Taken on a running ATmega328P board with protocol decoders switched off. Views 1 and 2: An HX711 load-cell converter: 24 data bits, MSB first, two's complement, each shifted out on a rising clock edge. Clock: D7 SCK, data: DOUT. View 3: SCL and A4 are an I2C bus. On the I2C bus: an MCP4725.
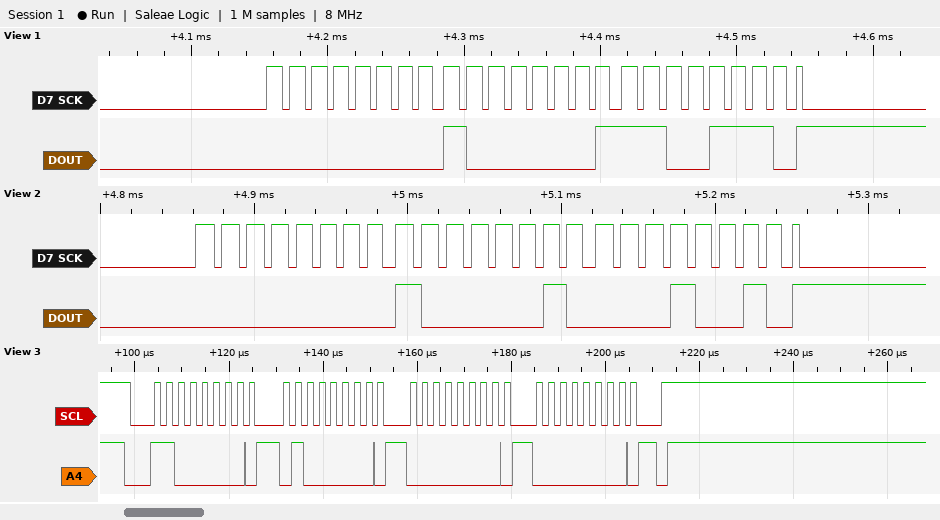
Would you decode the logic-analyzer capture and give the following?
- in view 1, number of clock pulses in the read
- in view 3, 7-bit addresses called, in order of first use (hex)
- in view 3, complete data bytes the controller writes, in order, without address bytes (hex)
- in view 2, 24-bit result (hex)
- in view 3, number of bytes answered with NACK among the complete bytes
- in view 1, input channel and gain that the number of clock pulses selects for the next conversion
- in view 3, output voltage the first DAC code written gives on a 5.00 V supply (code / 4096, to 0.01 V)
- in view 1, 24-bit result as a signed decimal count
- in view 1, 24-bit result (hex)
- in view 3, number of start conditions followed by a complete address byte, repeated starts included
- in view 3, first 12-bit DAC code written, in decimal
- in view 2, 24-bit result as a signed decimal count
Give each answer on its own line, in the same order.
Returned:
25
0x60
40 00 00
0x008212
0
channel A, gain 128
0.00 V
33230
0x0081CE
1
0
33298
